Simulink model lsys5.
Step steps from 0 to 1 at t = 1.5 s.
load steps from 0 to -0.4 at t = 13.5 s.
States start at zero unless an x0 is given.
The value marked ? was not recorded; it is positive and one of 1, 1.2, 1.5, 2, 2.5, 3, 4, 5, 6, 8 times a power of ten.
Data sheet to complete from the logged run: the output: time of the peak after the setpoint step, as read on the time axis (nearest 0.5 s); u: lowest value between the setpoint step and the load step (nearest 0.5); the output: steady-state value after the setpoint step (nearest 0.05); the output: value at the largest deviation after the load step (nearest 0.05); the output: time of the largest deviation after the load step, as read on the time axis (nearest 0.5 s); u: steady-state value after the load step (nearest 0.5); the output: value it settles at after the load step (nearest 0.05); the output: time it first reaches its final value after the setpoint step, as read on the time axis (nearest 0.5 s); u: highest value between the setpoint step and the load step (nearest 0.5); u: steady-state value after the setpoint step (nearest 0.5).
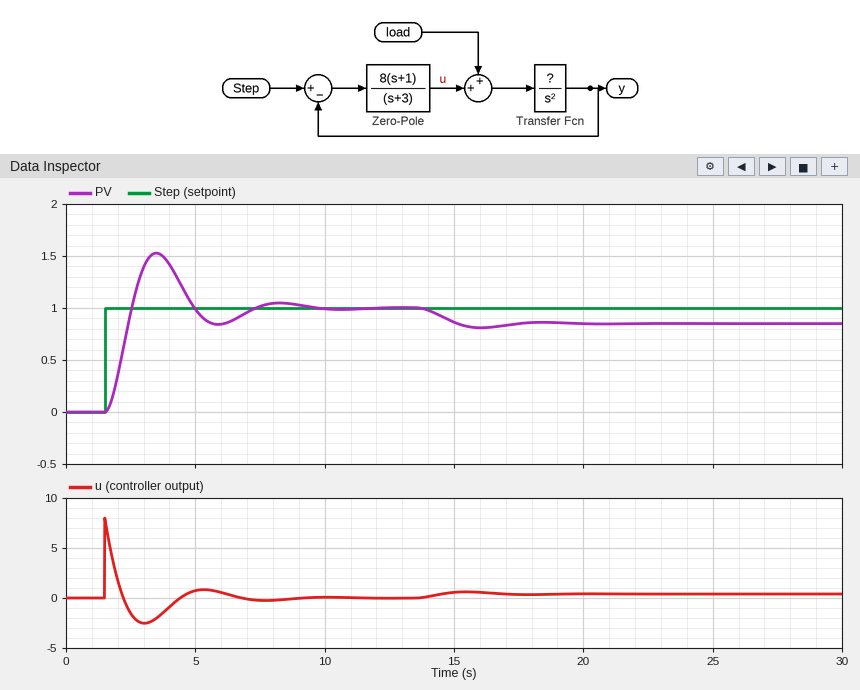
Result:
3.5 s
-2.5
1.00
0.80
16.0 s
0.5
0.85
2.5 s
8.0
0.0
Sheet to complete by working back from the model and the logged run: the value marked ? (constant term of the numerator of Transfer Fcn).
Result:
0.5
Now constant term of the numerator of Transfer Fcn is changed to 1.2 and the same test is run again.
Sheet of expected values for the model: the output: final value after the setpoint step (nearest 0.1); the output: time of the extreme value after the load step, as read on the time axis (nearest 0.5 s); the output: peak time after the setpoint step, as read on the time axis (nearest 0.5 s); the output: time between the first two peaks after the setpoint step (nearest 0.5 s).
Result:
1.0
15.0 s
2.5 s
2.5 s
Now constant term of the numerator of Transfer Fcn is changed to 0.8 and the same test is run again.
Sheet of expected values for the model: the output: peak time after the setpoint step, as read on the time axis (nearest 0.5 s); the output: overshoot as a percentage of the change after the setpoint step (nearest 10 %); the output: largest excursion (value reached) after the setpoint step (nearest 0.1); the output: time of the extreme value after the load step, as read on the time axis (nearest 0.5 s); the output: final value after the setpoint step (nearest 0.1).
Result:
3.0 s
50 %
1.5
15.5 s
1.0
